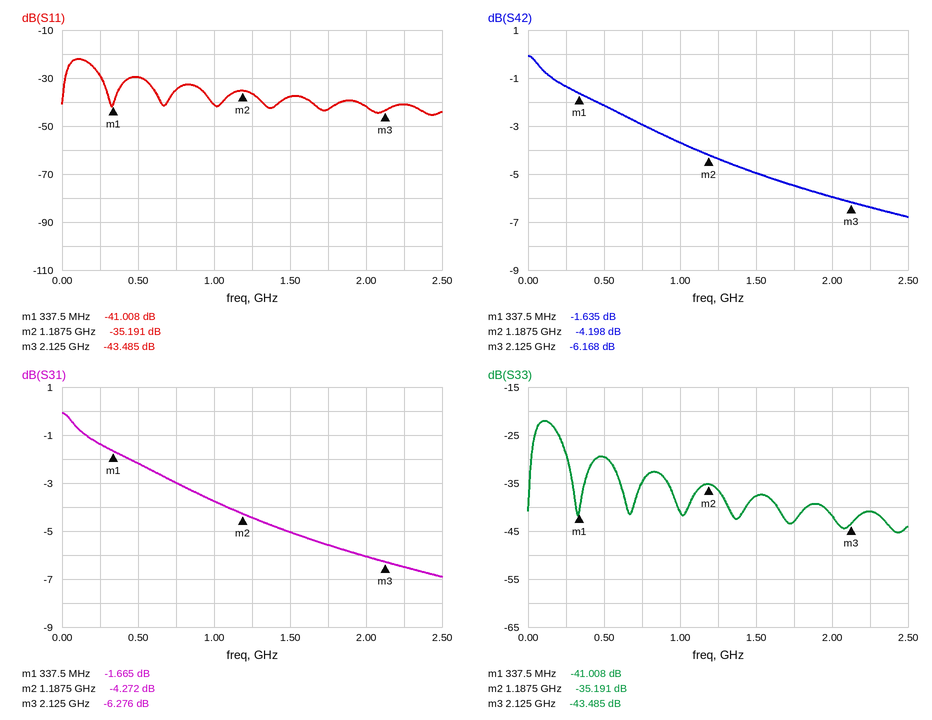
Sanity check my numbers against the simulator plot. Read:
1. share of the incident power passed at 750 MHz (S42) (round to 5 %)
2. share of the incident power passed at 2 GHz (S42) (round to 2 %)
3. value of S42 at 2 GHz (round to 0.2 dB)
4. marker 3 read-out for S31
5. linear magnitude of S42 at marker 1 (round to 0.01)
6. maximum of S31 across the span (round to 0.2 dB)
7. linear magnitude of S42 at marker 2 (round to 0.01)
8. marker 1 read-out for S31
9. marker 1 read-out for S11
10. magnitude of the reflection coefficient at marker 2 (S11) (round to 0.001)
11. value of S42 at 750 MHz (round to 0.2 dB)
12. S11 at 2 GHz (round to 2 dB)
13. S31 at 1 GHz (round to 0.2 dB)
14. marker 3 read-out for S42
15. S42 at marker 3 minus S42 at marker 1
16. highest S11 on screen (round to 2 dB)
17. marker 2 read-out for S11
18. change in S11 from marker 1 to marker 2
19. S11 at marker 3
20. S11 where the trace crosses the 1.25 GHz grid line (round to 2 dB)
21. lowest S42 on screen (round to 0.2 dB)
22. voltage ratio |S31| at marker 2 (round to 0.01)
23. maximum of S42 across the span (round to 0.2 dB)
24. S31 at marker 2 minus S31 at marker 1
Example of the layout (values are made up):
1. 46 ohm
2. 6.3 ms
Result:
1. 50 %
2. 26 %
3. -6.0 dB
4. -6.276 dB
5. 0.83
6. 0.0 dB
7. 0.62
8. -1.665 dB
9. -41.008 dB
10. 0.017
11. -3.0 dB
12. -42 dB
13. -3.8 dB
14. -6.168 dB
15. -4.533 dB
16. -22 dB
17. -35.191 dB
18. 5.817 dB
19. -43.485 dB
20. -36 dB
21. -6.8 dB
22. 0.61
23. 0.0 dB
24. -2.607 dB
